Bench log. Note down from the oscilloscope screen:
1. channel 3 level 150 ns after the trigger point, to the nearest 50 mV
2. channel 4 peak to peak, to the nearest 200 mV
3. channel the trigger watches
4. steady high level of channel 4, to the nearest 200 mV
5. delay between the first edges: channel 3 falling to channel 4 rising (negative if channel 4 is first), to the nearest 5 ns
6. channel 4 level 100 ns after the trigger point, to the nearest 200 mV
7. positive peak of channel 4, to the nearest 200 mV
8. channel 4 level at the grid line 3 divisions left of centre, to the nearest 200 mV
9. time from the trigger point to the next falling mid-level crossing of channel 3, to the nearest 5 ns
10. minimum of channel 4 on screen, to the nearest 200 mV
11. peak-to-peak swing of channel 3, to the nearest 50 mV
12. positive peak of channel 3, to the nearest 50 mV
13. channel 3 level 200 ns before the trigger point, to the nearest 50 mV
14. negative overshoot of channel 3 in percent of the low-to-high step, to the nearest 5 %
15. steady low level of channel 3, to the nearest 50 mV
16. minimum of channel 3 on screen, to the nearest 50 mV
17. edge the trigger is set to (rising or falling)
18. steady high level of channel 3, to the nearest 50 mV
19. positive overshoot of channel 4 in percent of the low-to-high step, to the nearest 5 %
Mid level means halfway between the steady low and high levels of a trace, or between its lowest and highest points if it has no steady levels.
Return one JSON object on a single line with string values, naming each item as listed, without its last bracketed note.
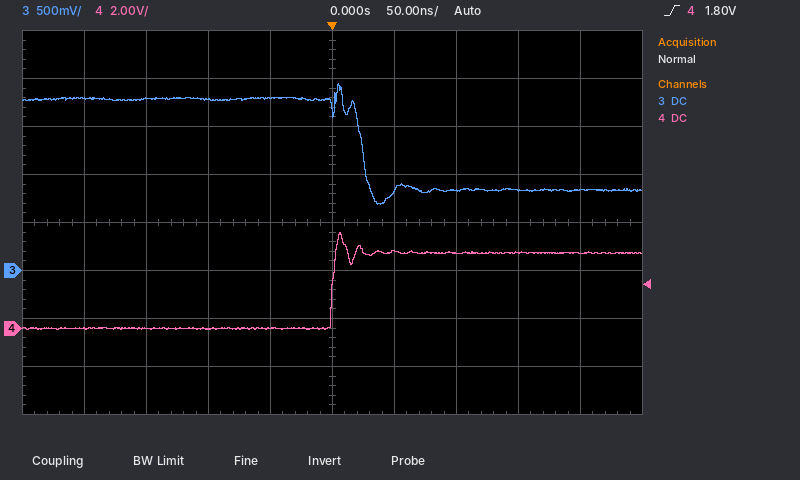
{"channel 3 level 150 ns after the trigger point, to the nearest 50 mV": "850 mV", "channel 4 peak to peak, to the nearest 200 mV": "4.0 V", "channel the trigger watches": "channel 4", "steady high level of channel 4, to the nearest 200 mV": "3.2 V", "delay between the first edges: channel 3 falling to channel 4 rising (negative if channel 4 is first), to the nearest 5 ns": "-25 ns", "channel 4 level 100 ns after the trigger point, to the nearest 200 mV": "3.2 V", "positive peak of channel 4, to the nearest 200 mV": "4.0 V", "channel 4 level at the grid line 3 divisions left of centre, to the nearest 200 mV": "0.0 V", "time from the trigger point to the next falling mid-level crossing of channel 3, to the nearest 5 ns": "25 ns", "minimum of channel 4 on screen, to the nearest 200 mV": "0.0 V", "peak-to-peak swing of channel 3, to the nearest 50 mV": "1.25 V", "positive peak of channel 3, to the nearest 50 mV": "1.95 V", "channel 3 level 200 ns before the trigger point, to the nearest 50 mV": "1.80 V", "negative overshoot of channel 3 in percent of the low-to-high step, to the nearest 5 %": "15 %", "steady low level of channel 3, to the nearest 50 mV": "850 mV", "minimum of channel 3 on screen, to the nearest 50 mV": "700 mV", "edge the trigger is set to": "rising", "steady high level of channel 3, to the nearest 50 mV": "1.80 V", "positive overshoot of channel 4 in percent of the low-to-high step, to the nearest 5 %": "25 %"}
